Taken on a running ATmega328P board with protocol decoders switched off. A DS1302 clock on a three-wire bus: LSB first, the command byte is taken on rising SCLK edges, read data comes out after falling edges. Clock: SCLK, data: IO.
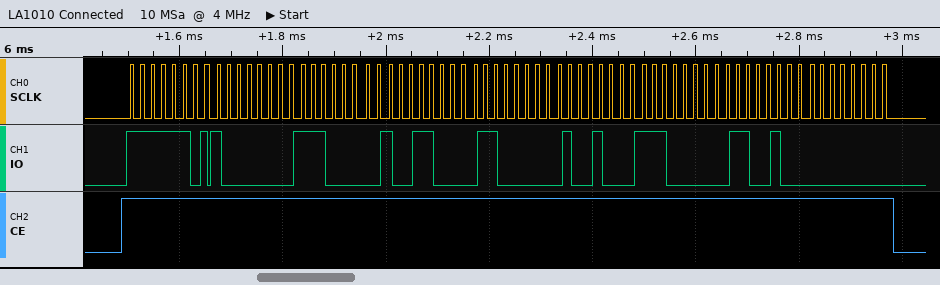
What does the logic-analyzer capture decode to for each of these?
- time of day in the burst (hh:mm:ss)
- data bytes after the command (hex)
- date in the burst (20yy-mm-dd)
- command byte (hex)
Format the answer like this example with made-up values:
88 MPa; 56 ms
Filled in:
19:07:01; 01 07 19 06 12 07 26 00; 2026-12-06; 0xBF
